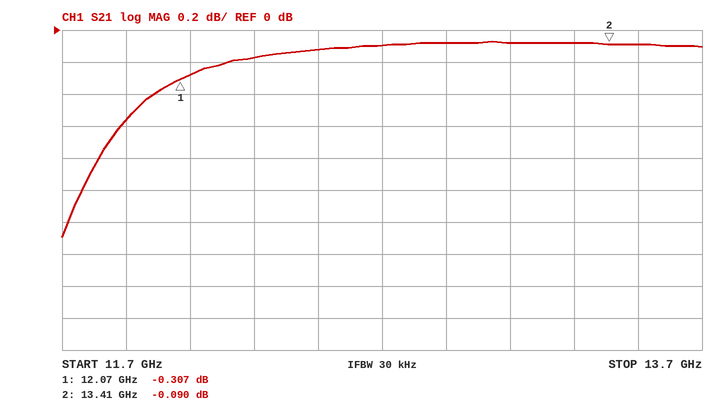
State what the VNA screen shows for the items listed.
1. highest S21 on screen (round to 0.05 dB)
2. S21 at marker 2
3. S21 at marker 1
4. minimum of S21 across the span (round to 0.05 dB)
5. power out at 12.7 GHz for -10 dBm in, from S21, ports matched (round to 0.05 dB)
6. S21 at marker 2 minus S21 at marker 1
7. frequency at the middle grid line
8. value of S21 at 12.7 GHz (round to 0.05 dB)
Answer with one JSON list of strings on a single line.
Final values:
["-0.05 dB", "-0.090 dB", "-0.307 dB", "-1.30 dB", "-10.10 dBm", "0.217 dB", "12.7 GHz", "-0.10 dB"]
